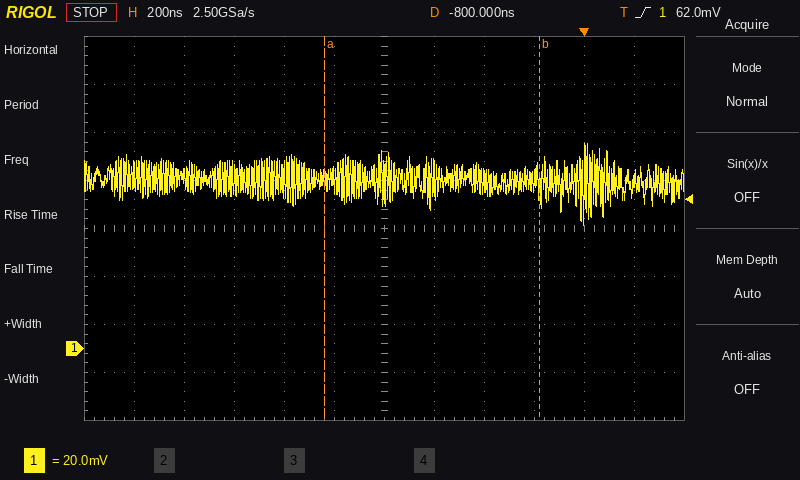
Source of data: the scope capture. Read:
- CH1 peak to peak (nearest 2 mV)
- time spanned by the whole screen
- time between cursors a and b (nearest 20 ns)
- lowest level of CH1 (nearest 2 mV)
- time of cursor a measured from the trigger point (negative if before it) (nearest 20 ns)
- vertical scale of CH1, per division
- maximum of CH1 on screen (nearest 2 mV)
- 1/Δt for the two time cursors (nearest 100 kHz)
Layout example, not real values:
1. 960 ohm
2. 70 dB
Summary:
1. 34 mV
2. 2.4 µs
3. 860 ns
4. 52 mV
5. -1.04 µs
6. 20 mV
7. 86 mV
8. 1.2 MHz
